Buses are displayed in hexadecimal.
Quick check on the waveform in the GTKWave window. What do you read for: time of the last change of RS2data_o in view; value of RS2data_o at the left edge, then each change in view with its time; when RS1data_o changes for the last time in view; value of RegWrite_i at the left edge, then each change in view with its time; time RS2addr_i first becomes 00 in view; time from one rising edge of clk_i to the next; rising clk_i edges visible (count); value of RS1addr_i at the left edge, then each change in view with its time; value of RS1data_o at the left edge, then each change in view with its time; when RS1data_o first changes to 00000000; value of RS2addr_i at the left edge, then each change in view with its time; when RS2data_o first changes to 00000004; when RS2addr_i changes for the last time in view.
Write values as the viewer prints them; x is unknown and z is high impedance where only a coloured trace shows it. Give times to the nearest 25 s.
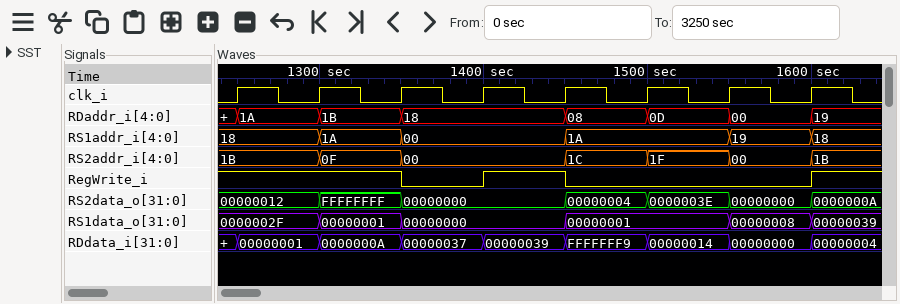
1600 s
00000012, FFFFFFFF at 1300 s, 00000000 at 1350 s, 00000004 at 1450 s, 0000003E at 1500 s, 00000000 at 1550 s, 0000000A at 1600 s
1600 s
1, 0 at 1350 s, 1 at 1400 s, 0 at 1450 s, 1 at 1600 s
1350 s
50 s
8
18, 1A at 1300 s, 00 at 1350 s, 1A at 1450 s, 19 at 1550 s, 18 at 1600 s
0000002F, 00000001 at 1300 s, 00000000 at 1350 s, 00000001 at 1450 s, 00000008 at 1550 s, 00000039 at 1600 s
1350 s
1B, 0F at 1300 s, 00 at 1350 s, 1C at 1450 s, 1F at 1500 s, 00 at 1550 s, 1B at 1600 s
1450 s
1600 s
